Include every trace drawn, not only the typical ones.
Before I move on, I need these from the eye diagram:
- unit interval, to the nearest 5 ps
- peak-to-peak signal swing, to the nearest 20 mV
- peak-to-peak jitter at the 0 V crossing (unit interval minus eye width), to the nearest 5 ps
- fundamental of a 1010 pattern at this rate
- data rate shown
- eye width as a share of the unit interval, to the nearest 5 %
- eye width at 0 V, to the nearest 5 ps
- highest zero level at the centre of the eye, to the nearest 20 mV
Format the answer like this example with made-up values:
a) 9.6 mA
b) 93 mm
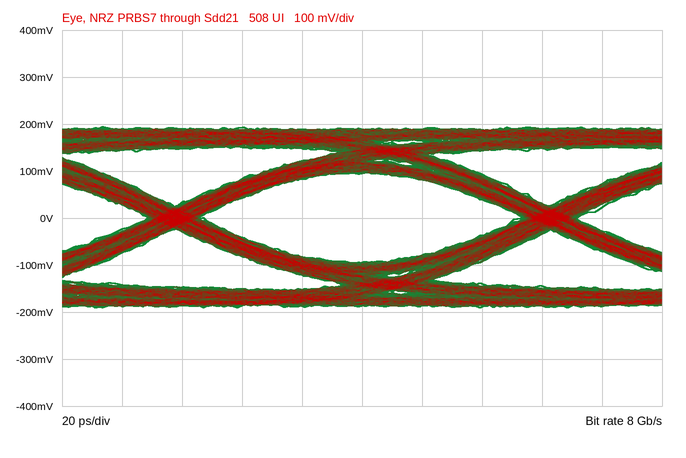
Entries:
a) 125 ps
b) 380 mV
c) 20 ps
d) 4 GHz
e) 8 Gb/s
f) 85 %
g) 105 ps
h) -100 mV
